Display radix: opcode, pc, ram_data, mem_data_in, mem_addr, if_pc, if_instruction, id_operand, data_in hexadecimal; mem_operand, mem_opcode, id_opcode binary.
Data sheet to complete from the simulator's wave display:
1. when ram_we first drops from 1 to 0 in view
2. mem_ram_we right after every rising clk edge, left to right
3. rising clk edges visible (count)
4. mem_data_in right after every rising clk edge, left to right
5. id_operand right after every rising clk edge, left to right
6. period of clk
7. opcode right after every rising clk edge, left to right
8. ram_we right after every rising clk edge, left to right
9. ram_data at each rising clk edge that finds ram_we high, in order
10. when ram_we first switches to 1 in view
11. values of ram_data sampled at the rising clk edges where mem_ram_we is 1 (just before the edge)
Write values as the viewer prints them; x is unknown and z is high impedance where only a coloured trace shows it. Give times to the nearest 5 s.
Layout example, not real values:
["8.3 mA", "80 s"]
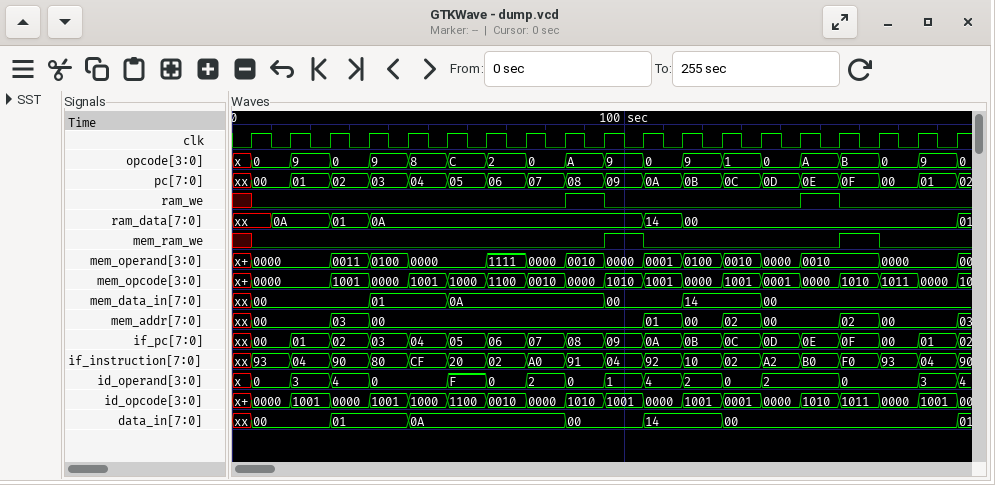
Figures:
["95 s", "0 0 0 0 0 0 0 0 0 1 0 0 0 0 0 1 0 0 0", "19", "00, 00, 00, 01, 01, 0A, 0A, 0A, 0A, 00, 00, 14, 14, 00, 00, 00, 00, 00, 00", "0, 3, 4, 0, 0, F, 0, 2, 0, 1, 4, 2, 0, 2, 2, 0, 0, 3, 4", "10 s", "0, 9, 0, 9, 8, C, 2, 0, A, 9, 0, 9, 1, 0, A, B, 0, 9, 0", "0 0 0 0 0 0 0 0 1 0 0 0 0 0 1 0 0 0 0", "0A, 00", "85 s", "0A, 00"]
